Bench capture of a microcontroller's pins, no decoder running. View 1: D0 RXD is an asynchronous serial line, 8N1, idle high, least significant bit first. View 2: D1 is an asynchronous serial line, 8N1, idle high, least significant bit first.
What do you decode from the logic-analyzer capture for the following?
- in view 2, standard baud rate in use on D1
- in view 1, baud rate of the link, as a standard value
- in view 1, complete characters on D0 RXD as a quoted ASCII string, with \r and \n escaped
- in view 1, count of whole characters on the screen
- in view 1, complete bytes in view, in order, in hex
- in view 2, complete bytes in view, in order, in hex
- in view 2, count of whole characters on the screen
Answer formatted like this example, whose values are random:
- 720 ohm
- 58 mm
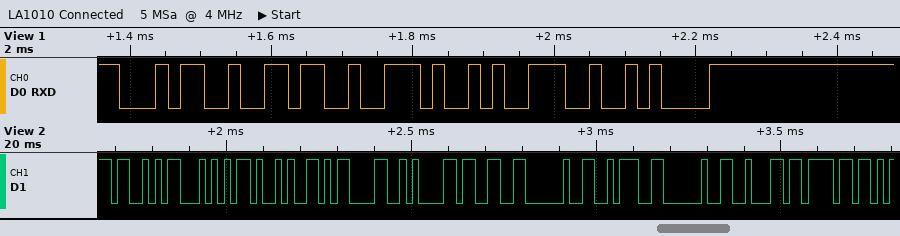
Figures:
- 57600 baud
- 57600 baud
- "46.9\n"
- 5
- 0x34 0x36 0x2E 0x39 0x0A
- 0x53 0x54 0x29 0x0D 0x0A 0x33 0x20 0x3A 0x20 0x62 0x6F
- 11
